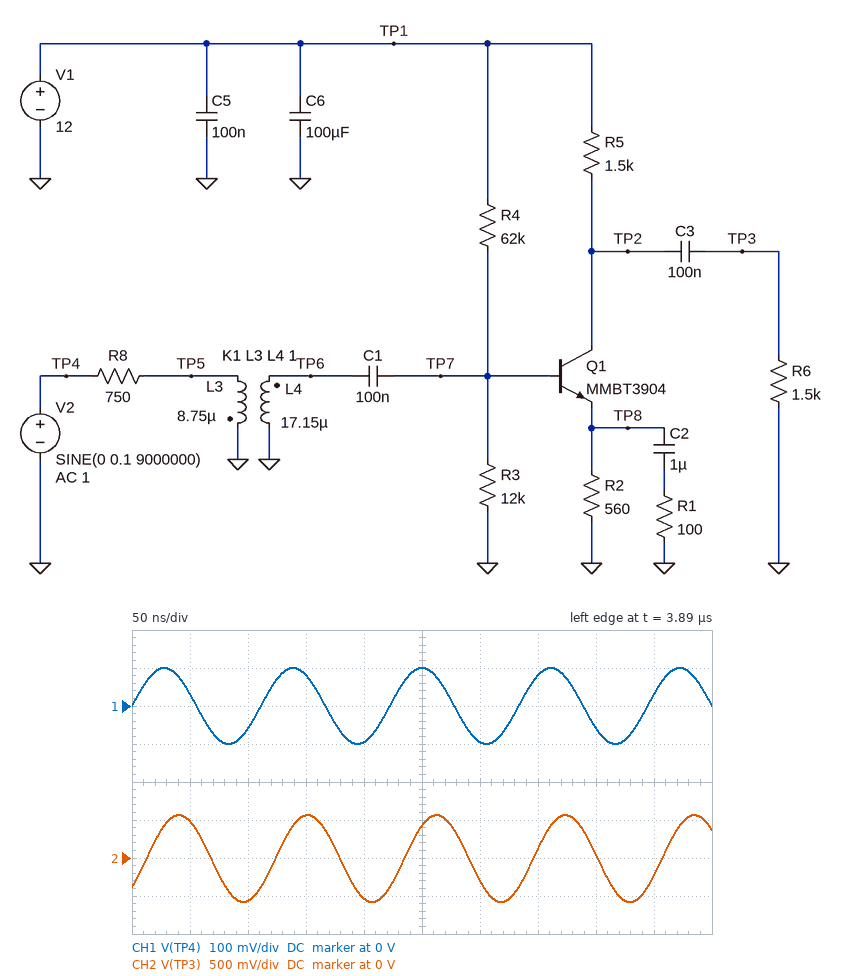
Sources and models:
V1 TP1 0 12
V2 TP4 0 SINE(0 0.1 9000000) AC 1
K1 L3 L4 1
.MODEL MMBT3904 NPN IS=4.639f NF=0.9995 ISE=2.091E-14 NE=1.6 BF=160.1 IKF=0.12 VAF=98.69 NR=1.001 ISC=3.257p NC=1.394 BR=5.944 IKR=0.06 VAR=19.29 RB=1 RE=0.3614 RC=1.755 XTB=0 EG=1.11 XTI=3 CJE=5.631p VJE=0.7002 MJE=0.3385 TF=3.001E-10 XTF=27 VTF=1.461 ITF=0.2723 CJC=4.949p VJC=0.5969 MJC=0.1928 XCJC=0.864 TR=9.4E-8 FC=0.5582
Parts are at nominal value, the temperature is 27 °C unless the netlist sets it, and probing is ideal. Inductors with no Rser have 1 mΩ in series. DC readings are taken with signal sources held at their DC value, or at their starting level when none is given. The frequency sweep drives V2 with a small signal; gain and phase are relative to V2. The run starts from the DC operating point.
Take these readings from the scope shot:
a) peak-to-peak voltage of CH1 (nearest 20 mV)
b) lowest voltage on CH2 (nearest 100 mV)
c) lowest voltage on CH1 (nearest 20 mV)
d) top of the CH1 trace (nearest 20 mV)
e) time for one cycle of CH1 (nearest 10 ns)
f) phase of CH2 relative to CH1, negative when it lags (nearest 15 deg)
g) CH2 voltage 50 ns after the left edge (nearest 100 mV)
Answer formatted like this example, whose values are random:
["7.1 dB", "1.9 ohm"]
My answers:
["200 mV", "-600 mV", "-100 mV", "100 mV", "110 ns", "-45 deg", "500 mV"]
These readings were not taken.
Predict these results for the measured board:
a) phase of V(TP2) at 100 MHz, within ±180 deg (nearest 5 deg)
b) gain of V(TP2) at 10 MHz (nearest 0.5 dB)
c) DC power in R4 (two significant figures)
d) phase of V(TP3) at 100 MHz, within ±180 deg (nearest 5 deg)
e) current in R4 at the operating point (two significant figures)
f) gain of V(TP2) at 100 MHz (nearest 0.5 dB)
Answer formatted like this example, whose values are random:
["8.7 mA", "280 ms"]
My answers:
["-110 deg", "14.0 dB", "1.7 mW", "-110 deg", "160 µA", "-8.5 dB"]
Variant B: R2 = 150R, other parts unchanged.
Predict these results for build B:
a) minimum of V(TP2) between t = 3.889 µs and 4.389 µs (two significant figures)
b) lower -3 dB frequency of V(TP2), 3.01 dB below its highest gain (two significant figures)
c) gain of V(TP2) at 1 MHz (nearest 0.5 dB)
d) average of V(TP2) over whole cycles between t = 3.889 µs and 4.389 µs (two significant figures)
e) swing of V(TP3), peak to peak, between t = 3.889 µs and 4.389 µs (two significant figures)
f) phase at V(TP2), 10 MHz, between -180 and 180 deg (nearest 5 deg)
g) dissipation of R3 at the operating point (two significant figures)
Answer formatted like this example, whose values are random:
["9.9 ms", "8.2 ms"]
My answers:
["3.2 V", "3.9 MHz", "1.5 dB", "3.6 V", "950 mV", "-70 deg", "200 µW"]
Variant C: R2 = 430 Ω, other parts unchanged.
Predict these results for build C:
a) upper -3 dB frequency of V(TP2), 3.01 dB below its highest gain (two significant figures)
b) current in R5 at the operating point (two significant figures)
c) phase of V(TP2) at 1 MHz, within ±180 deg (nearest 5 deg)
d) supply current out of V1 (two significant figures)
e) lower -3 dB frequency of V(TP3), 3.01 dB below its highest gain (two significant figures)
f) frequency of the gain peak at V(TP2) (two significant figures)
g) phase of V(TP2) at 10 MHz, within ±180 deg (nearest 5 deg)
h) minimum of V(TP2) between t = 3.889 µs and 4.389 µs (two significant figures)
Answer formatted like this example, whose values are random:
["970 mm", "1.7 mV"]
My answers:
["9.2 MHz", "2.5 mA", "85 deg", "2.7 mA", "4.7 MHz", "6.6 MHz", "-55 deg", "7.7 V"]
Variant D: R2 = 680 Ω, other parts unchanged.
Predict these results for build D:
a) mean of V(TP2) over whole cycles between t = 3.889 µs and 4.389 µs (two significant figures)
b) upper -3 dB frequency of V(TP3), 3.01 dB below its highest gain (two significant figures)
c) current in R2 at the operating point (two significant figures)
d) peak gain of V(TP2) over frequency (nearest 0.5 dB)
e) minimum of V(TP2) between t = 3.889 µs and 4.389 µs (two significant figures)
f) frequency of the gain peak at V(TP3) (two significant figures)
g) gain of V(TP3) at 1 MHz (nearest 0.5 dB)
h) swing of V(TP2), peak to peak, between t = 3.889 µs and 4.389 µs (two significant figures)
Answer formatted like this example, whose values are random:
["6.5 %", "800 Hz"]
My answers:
["9.5 V", "9.9 MHz", "1.7 mA", "17.0 dB", "8.9 V", "6.9 MHz", "-2.5 dB", "1.1 V"]
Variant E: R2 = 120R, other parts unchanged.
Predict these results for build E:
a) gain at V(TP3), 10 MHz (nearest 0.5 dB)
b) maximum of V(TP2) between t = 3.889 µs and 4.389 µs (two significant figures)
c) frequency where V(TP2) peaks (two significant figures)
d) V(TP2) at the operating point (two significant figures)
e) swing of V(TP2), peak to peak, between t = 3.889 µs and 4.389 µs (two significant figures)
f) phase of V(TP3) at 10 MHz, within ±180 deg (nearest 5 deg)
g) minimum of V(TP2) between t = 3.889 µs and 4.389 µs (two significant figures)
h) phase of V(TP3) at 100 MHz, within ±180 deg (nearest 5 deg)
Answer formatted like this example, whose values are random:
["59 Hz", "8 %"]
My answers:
["11.0 dB", "2.8 V", "4.8 MHz", "2.4 V", "830 mV", "-75 deg", "2.0 V", "-110 deg"]
